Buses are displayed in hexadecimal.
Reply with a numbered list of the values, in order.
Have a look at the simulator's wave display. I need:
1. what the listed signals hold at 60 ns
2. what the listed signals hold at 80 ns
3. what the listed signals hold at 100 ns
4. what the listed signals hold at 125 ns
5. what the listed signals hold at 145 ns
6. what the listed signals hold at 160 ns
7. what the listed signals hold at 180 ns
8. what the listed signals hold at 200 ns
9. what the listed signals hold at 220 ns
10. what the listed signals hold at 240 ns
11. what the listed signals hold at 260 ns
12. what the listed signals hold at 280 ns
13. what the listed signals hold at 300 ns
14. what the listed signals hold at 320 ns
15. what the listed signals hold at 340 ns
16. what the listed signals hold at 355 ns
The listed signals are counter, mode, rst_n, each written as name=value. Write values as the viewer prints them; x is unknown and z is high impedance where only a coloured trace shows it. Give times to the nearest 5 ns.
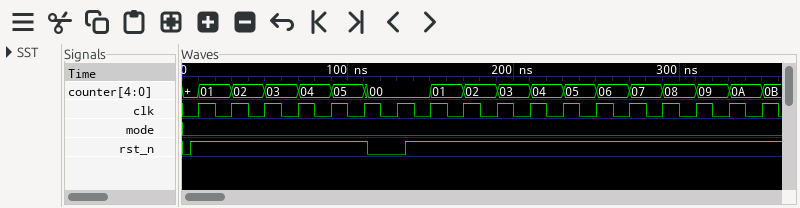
1. counter=03, mode=0, rst_n=1
2. counter=04, mode=0, rst_n=1
3. counter=05, mode=0, rst_n=1
4. counter=00, mode=0, rst_n=0
5. counter=00, mode=0, rst_n=1
6. counter=01, mode=0, rst_n=1
7. counter=02, mode=0, rst_n=1
8. counter=03, mode=0, rst_n=1
9. counter=04, mode=0, rst_n=1
10. counter=05, mode=0, rst_n=1
11. counter=06, mode=0, rst_n=1
12. counter=07, mode=0, rst_n=1
13. counter=08, mode=0, rst_n=1
14. counter=09, mode=0, rst_n=1
15. counter=0A, mode=0, rst_n=1
16. counter=0B, mode=0, rst_n=1
